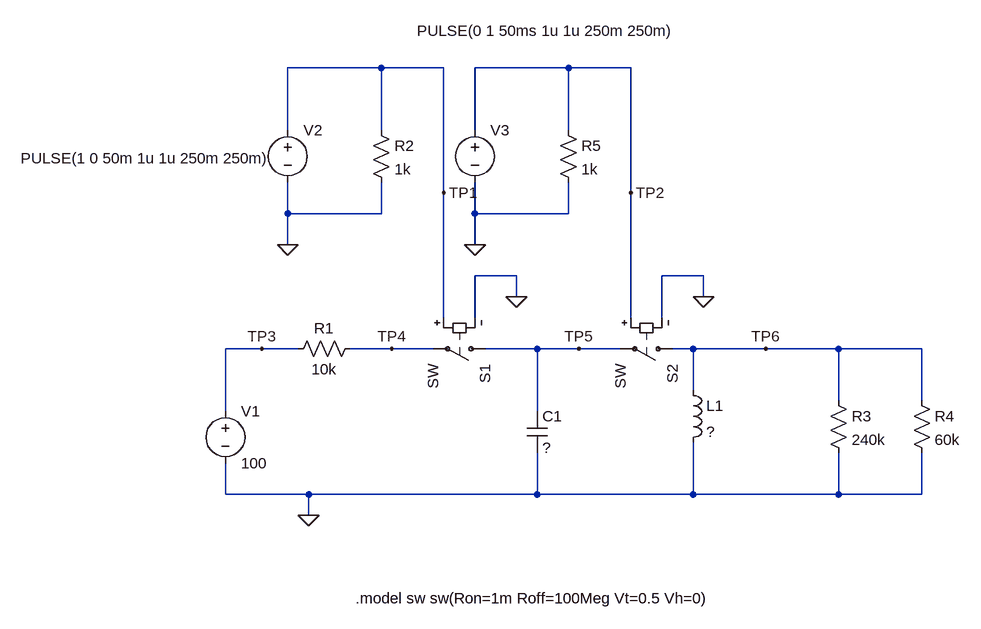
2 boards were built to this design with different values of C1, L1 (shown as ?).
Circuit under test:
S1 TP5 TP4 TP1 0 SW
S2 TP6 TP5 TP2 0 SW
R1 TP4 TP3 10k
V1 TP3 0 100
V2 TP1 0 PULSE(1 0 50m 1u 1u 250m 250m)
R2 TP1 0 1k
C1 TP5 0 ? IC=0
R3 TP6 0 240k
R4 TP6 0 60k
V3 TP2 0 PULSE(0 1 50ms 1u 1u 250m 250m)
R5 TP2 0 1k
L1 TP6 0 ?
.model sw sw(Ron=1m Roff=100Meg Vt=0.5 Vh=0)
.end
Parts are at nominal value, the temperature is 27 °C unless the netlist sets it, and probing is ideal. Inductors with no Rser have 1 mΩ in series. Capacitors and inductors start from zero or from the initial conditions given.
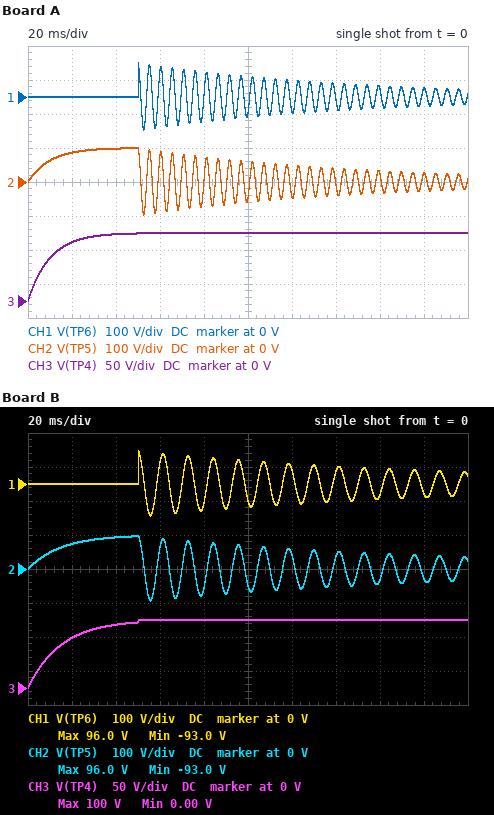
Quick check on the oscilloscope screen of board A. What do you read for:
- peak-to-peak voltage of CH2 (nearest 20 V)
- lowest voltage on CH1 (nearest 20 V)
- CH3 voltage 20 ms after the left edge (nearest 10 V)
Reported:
200 V
-100 V
90 V
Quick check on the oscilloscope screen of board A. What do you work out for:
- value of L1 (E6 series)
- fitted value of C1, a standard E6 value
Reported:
680 mH
1 µF
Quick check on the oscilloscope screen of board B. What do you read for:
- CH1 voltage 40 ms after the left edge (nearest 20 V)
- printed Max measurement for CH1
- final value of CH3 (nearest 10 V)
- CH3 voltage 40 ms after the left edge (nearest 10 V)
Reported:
0 V
96.0 V
100 V
90 V
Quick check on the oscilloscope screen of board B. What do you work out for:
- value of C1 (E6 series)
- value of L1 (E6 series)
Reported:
1.5 µF
2.2 H
